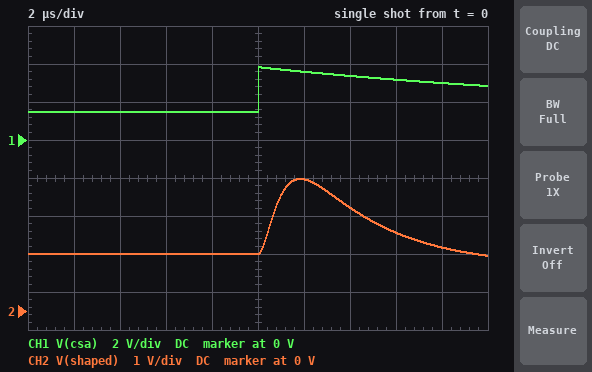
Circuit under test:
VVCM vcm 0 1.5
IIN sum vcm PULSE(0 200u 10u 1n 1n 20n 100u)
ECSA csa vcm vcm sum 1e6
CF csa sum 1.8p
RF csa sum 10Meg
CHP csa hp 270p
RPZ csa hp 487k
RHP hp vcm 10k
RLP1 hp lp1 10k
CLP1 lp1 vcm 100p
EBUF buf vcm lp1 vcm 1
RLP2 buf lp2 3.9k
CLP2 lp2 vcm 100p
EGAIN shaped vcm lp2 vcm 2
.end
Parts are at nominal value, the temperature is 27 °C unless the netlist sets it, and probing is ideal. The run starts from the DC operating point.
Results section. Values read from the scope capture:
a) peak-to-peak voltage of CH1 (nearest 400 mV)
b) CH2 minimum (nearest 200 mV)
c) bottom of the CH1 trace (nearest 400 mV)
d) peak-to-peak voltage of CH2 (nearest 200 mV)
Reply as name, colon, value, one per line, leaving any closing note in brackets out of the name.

peak-to-peak voltage of CH1: 2.4 V
CH2 minimum: 1.4 V
bottom of the CH1 trace: 1.6 V
peak-to-peak voltage of CH2: 2.0 V
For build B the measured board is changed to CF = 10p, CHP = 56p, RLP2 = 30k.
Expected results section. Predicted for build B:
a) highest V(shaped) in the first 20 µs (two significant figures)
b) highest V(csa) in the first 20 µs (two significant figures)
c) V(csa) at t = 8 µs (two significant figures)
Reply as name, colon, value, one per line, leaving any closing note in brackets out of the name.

highest V(shaped) in the first 20 µs: 1.6 V
highest V(csa) in the first 20 µs: 1.9 V
V(csa) at t = 8 µs: 1.5 V
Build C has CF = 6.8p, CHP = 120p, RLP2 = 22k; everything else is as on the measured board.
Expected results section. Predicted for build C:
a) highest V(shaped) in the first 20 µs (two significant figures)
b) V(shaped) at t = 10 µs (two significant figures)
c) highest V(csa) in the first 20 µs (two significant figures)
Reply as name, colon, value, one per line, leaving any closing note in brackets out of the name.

highest V(shaped) in the first 20 µs: 1.7 V
V(shaped) at t = 10 µs: 1.5 V
highest V(csa) in the first 20 µs: 2.1 V
